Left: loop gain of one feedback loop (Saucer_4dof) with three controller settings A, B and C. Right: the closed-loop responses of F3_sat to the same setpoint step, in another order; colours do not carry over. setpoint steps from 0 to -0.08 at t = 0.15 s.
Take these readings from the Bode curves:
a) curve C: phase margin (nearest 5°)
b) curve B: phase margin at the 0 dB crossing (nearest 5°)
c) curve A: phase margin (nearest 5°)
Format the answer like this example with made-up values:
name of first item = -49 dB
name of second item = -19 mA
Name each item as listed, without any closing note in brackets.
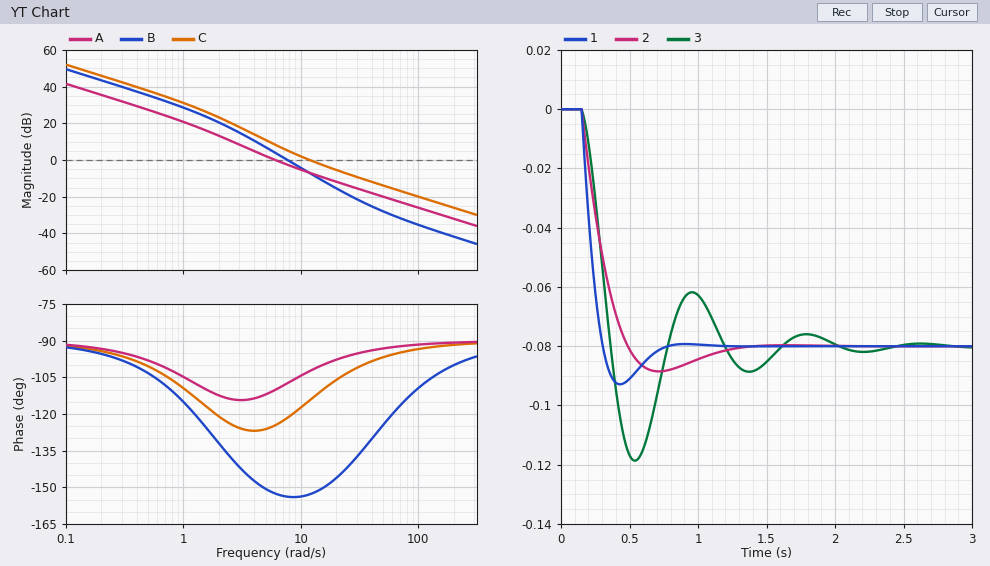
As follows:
curve C: phase margin = 65°
curve B: phase margin at the 0 dB crossing = 25°
curve A: phase margin = 70°
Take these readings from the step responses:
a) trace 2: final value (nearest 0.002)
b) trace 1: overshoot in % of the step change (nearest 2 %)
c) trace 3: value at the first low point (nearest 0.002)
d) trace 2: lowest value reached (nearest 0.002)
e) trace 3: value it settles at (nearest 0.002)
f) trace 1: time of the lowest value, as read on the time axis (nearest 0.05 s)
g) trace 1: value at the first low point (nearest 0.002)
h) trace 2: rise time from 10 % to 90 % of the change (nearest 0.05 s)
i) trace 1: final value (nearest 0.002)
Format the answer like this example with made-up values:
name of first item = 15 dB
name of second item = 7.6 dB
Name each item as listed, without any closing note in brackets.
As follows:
trace 2: final value = -0.080
trace 1: overshoot in % of the step change = 16 %
trace 3: value at the first low point = -0.118
trace 2: lowest value reached = -0.088
trace 3: value it settles at = -0.080
trace 1: time of the lowest value, as read on the time axis = 0.45 s
trace 1: value at the first low point = -0.092
trace 2: rise time from 10 % to 90 % of the change = 0.25 s
trace 1: final value = -0.080
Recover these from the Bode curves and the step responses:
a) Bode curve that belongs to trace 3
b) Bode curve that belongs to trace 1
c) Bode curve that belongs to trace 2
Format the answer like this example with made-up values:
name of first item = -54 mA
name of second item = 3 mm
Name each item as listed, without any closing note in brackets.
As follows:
Bode curve that belongs to trace 3 = B
Bode curve that belongs to trace 1 = C
Bode curve that belongs to trace 2 = A
